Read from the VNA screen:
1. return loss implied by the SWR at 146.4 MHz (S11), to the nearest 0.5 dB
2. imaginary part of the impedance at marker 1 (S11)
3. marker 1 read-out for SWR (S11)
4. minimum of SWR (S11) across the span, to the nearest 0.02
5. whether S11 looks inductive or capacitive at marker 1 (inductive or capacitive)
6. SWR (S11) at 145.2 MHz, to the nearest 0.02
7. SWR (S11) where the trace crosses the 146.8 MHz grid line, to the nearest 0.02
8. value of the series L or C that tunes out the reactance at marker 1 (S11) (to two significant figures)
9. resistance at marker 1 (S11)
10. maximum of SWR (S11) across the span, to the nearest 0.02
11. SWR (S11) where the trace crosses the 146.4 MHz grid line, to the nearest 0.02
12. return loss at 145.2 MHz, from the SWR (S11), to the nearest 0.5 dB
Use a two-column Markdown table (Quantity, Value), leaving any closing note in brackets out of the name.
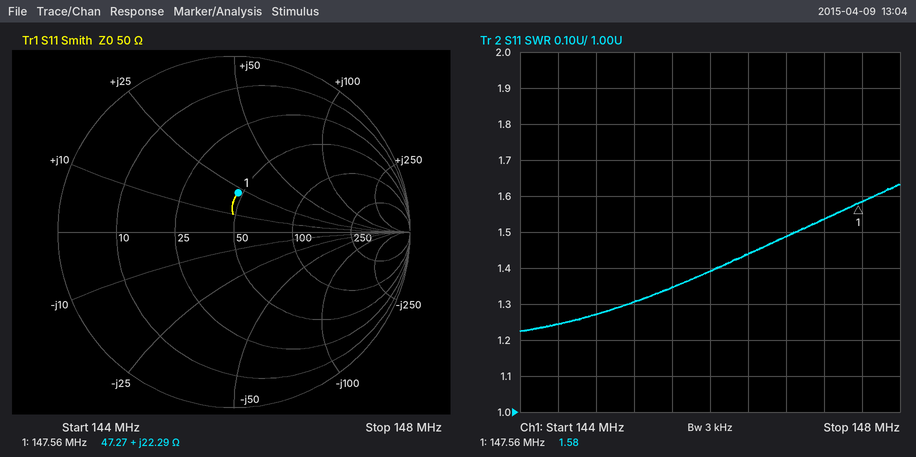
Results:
| Quantity | Value |
|---|---|
| return loss implied by the SWR at 146.4 MHz (S11), to the nearest 0.5 dB | 15.0 dB |
| imaginary part of the impedance at marker 1 | +22.29 Ω |
| marker 1 read-out for SWR | 1.58 |
| minimum of SWR (S11) across the span, to the nearest 0.02 | 1.22 |
| whether S11 looks inductive or capacitive at marker 1 | inductive |
| SWR (S11) at 145.2 MHz, to the nearest 0.02 | 1.30 |
| SWR (S11) where the trace crosses the 146.8 MHz grid line, to the nearest 0.02 | 1.48 |
| value of the series L or C that tunes out the reactance at marker 1 (S11) | 48 pF |
| resistance at marker 1 | 47.27 Ω |
| maximum of SWR (S11) across the span, to the nearest 0.02 | 1.64 |
| SWR (S11) where the trace crosses the 146.4 MHz grid line, to the nearest 0.02 | 1.44 |
| return loss at 145.2 MHz, from the SWR (S11), to the nearest 0.5 dB | 17.5 dB |
